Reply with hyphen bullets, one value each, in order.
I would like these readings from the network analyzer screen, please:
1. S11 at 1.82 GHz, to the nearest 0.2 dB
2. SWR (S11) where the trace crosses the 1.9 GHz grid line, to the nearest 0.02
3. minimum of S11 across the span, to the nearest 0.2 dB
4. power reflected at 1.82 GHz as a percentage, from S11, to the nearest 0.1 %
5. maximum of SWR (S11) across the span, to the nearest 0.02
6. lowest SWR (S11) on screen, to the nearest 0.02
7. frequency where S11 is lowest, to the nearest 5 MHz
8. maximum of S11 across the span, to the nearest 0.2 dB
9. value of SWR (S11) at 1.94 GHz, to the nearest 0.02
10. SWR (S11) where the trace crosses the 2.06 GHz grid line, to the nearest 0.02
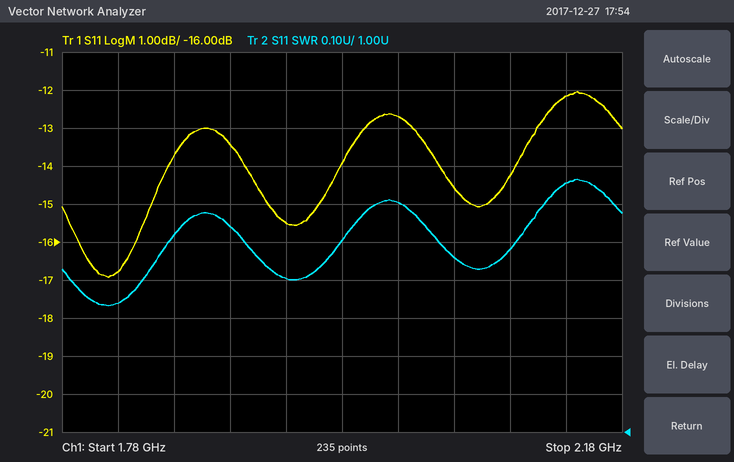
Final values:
- -16.8 dB
- 1.54
- -17.0 dB
- 2.1 %
- 1.66
- 1.34
- 1.815 GHz
- -12.0 dB
- 1.40
- 1.46
